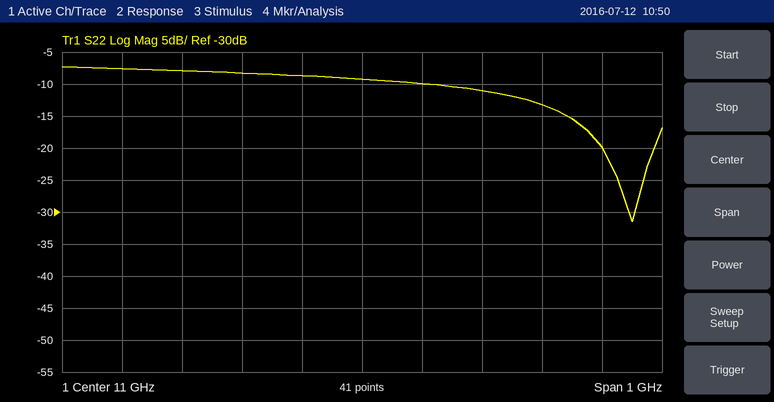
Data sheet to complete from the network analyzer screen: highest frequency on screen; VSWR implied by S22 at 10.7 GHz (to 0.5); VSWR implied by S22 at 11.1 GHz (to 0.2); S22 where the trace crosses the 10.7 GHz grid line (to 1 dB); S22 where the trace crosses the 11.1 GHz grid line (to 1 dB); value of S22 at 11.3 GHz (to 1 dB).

11.5 GHz
2.5
2.0
-8 dB
-10 dB
-13 dB
